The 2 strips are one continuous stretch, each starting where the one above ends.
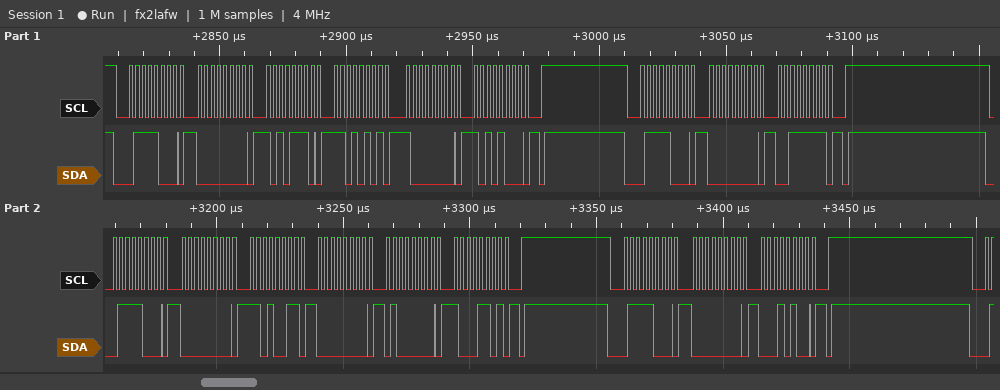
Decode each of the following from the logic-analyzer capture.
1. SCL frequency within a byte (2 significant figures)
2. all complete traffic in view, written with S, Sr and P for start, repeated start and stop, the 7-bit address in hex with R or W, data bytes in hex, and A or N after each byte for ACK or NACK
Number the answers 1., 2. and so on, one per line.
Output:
1. 400 kHz
2. S 3CW A 00 A AE A D5 A 80 A A8 A P S 3CW A 00 A 3F A P S 3CW A 00 A D3 A 00 A 40 A 8D A P S 3CW A 00 A 14 A P
